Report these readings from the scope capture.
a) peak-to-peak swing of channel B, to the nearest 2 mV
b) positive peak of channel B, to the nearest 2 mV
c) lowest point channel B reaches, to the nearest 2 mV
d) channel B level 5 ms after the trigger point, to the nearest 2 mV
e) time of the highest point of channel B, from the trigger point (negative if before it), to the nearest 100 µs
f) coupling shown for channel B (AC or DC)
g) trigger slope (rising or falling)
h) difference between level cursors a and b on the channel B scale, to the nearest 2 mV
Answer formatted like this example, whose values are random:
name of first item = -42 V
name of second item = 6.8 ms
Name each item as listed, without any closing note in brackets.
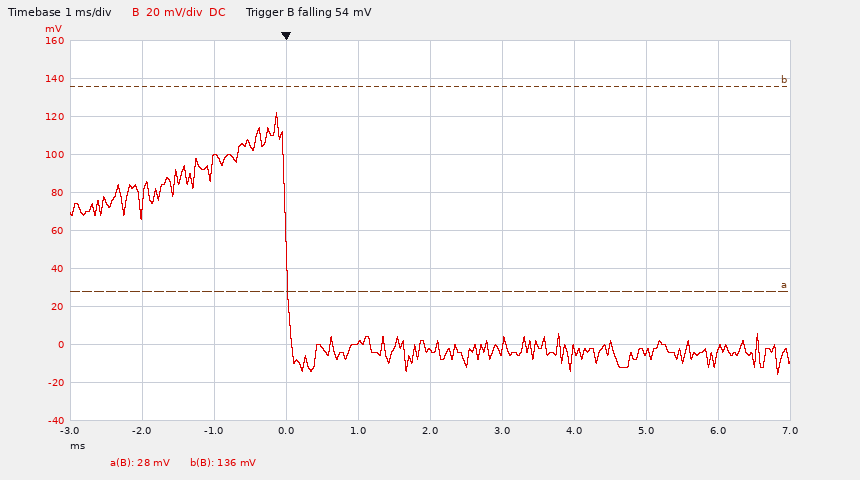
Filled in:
peak-to-peak swing of channel B, to the nearest 2 mV = 138 mV
positive peak of channel B, to the nearest 2 mV = 122 mV
lowest point channel B reaches, to the nearest 2 mV = -16 mV
channel B level 5 ms after the trigger point, to the nearest 2 mV = -4 mV
time of the highest point of channel B, from the trigger point (negative if before it), to the nearest 100 µs = -100 µs
coupling shown for channel B = DC
trigger slope = falling
difference between level cursors a and b on the channel B scale, to the nearest 2 mV = 108 mV
